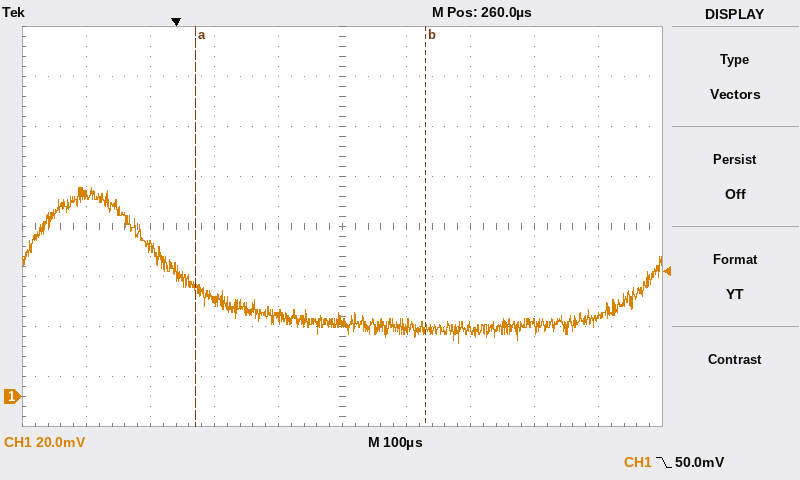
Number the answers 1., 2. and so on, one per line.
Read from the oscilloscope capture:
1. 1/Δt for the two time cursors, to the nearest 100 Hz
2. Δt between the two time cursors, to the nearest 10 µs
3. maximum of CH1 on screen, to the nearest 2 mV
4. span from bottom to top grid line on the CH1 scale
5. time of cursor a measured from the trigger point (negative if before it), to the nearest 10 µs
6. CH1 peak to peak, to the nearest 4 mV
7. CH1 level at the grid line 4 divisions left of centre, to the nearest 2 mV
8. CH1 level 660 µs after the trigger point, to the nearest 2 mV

1. 2.8 kHz
2. 360 µs
3. 84 mV
4. 160 mV
5. +30 µs
6. 64 mV
7. 80 mV
8. 32 mV
